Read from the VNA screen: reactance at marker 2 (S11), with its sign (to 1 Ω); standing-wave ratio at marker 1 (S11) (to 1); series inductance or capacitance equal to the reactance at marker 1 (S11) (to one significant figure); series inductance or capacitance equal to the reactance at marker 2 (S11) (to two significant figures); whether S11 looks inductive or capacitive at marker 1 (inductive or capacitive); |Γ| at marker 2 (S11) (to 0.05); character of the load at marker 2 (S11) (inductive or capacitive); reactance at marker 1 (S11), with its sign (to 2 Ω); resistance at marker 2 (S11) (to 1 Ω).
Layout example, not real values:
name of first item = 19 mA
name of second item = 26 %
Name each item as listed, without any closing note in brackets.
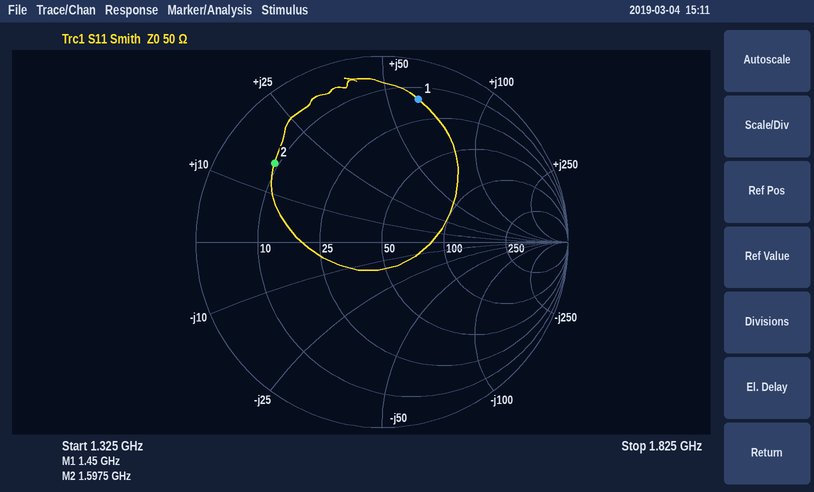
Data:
reactance at marker 2 (S11), with its sign = +16 Ω
standing-wave ratio at marker 1 (S11) = 9
series inductance or capacitance equal to the reactance at marker 1 (S11) = 7 nH
series inductance or capacitance equal to the reactance at marker 2 (S11) = 1.6 nH
whether S11 looks inductive or capacitive at marker 1 = inductive
|Γ| at marker 2 (S11) = 0.70
character of the load at marker 2 (S11) = inductive
reactance at marker 1 (S11), with its sign = +62 Ω
resistance at marker 2 (S11) = 9 Ω
